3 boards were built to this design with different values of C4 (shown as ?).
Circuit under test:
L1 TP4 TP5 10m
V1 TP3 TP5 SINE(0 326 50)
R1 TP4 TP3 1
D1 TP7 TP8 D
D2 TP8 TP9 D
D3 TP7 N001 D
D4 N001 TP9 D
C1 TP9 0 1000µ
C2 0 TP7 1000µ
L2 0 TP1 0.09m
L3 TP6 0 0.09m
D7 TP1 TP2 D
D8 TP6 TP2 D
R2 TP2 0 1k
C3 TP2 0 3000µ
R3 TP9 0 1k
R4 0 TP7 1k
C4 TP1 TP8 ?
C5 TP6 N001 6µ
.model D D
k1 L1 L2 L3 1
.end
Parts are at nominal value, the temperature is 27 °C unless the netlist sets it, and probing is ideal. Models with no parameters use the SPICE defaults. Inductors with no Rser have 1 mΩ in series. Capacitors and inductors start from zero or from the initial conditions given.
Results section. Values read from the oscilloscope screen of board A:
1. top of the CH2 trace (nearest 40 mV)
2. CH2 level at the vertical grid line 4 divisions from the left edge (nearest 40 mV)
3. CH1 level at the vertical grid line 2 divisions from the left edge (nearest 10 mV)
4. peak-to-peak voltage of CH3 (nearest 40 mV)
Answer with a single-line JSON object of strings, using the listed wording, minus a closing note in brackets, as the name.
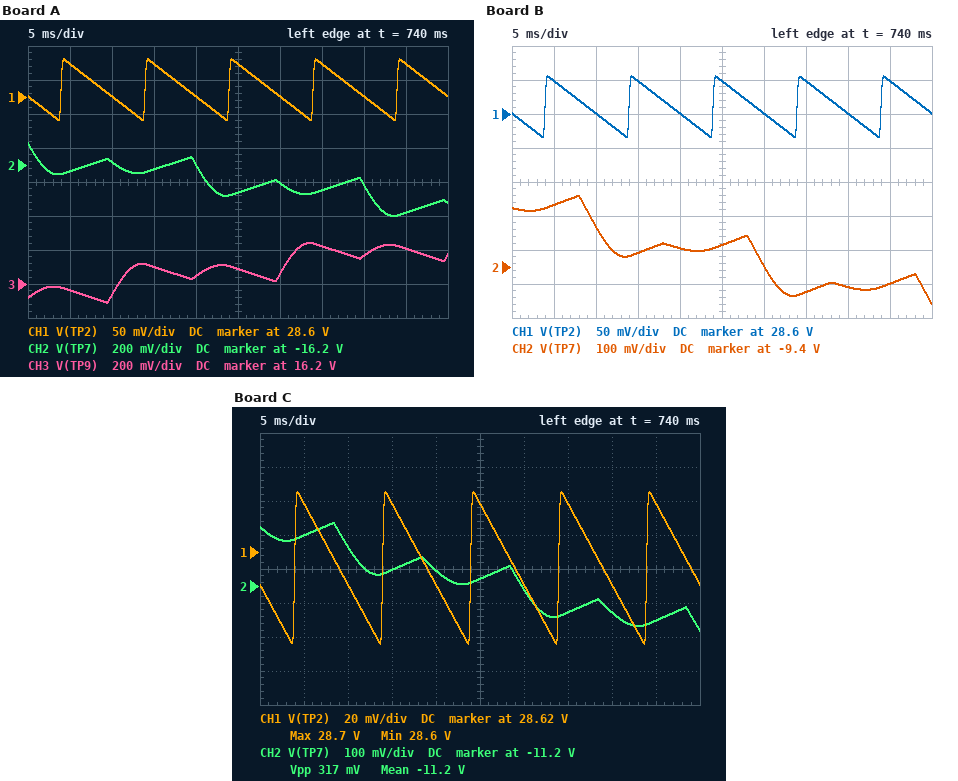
{"top of the CH2 trace": "-16.08 V", "CH2 level at the vertical grid line 4 divisions from the left edge": "-16.20 V", "CH1 level at the vertical grid line 2 divisions from the left edge": "28.60 V", "peak-to-peak voltage of CH3": "360 mV"}
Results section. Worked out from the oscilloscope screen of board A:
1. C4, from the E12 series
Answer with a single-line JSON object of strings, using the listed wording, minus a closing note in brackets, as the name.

{"C4, from the E12 series": "12 µF"}
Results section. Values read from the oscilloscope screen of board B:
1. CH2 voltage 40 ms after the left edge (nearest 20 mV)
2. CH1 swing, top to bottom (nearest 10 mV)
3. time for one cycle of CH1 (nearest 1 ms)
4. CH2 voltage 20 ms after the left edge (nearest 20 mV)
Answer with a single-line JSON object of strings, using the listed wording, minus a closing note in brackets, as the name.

{"CH2 voltage 40 ms after the left edge": "-9.46 V", "CH1 swing, top to bottom": "90 mV", "time for one cycle of CH1": "10 ms", "CH2 voltage 20 ms after the left edge": "-9.34 V"}
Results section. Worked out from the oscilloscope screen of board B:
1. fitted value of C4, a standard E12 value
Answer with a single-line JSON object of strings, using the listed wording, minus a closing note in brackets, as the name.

{"fitted value of C4, a standard E12 value": "1.8 µF"}
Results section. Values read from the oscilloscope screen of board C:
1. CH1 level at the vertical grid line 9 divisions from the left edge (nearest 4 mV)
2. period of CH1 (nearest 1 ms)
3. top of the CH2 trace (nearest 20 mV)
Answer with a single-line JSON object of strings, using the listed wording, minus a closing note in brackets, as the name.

{"CH1 level at the vertical grid line 9 divisions from the left edge": "28.648 V", "period of CH1": "10 ms", "top of the CH2 trace": "-11.02 V"}
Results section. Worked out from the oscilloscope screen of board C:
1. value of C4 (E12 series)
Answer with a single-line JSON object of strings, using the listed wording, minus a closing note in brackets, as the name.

{"value of C4": "3.9 µF"}
